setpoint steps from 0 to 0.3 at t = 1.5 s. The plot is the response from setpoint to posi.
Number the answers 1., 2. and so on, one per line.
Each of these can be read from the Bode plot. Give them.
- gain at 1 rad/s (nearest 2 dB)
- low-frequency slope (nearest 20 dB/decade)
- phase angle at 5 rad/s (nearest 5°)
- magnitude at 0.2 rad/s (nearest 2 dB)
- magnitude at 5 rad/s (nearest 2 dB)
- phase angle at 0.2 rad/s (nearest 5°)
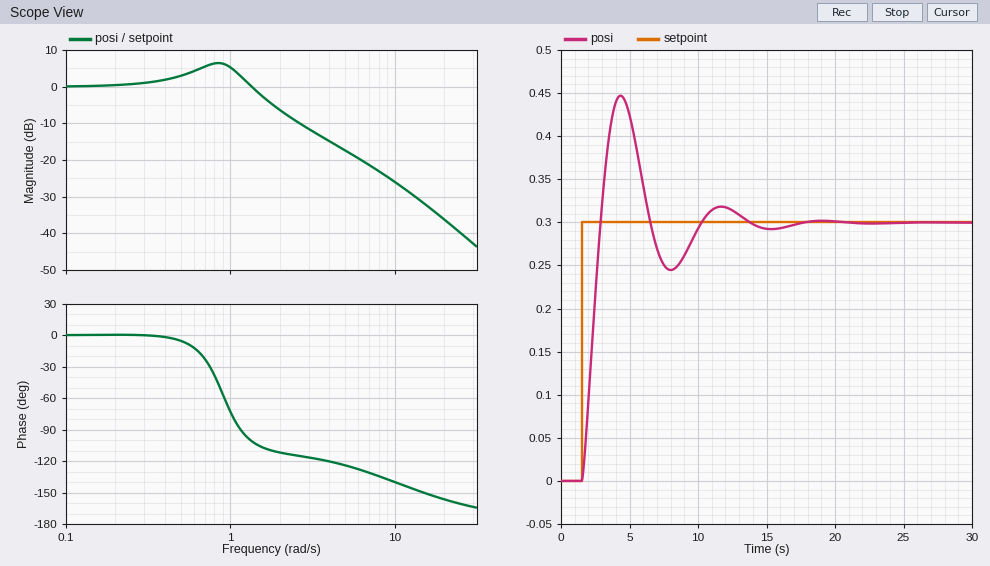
1. 6 dB
2. 0 dB/decade
3. -125°
4. 0 dB
5. -18 dB
6. 0°
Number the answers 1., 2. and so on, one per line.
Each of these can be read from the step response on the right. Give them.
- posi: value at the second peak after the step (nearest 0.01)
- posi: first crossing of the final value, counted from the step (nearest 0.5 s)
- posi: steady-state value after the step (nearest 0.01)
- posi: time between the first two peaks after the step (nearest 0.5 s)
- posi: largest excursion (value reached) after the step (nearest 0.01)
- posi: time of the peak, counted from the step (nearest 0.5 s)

1. 0.32
2. 1.5 s
3. 0.30
4. 7.5 s
5. 0.45
6. 3.0 s
